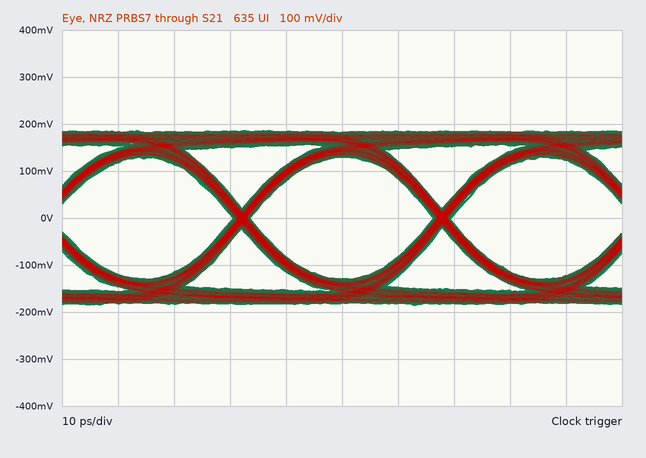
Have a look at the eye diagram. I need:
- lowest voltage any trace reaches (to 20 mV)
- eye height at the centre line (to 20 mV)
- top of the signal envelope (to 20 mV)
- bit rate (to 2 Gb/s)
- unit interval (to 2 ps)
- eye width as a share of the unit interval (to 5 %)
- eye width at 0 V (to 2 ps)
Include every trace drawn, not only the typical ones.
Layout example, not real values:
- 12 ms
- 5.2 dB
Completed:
- -180 mV
- 260 mV
- 180 mV
- 28 Gb/s
- 36 ps
- 90 %
- 32 ps
